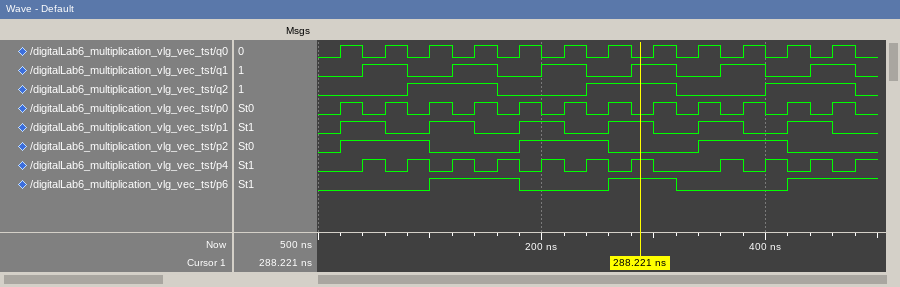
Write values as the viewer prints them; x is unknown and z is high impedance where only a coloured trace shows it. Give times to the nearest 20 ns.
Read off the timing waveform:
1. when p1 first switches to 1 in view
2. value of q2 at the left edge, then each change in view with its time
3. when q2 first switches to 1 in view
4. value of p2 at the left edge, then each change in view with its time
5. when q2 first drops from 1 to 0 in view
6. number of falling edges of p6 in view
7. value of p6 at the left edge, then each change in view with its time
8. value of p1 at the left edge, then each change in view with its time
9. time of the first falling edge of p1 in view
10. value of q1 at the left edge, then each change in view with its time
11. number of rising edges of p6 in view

20 ns
0, 1 at 80 ns, 0 at 160 ns, 1 at 240 ns, 0 at 320 ns, 1 at 400 ns, 0 at 480 ns
80 ns
0, 1 at 20 ns, 0 at 100 ns, 1 at 180 ns, 0 at 260 ns, 1 at 340 ns, 0 at 420 ns
160 ns
2
0, 1 at 100 ns, 0 at 180 ns, 1 at 260 ns, 0 at 320 ns, 1 at 420 ns
0, 1 at 20 ns, 0 at 60 ns, 1 at 100 ns, 0 at 140 ns, 1 at 180 ns, 0 at 220 ns, 1 at 260 ns, 0 at 300 ns, 1 at 340 ns, 0 at 380 ns, 1 at 420 ns, 0 at 460 ns
60 ns
0, 1 at 40 ns, 0 at 80 ns, 1 at 120 ns, 0 at 160 ns, 1 at 200 ns, 0 at 240 ns, 1 at 280 ns, 0 at 320 ns, 1 at 360 ns, 0 at 400 ns, 1 at 440 ns, 0 at 480 ns
3
